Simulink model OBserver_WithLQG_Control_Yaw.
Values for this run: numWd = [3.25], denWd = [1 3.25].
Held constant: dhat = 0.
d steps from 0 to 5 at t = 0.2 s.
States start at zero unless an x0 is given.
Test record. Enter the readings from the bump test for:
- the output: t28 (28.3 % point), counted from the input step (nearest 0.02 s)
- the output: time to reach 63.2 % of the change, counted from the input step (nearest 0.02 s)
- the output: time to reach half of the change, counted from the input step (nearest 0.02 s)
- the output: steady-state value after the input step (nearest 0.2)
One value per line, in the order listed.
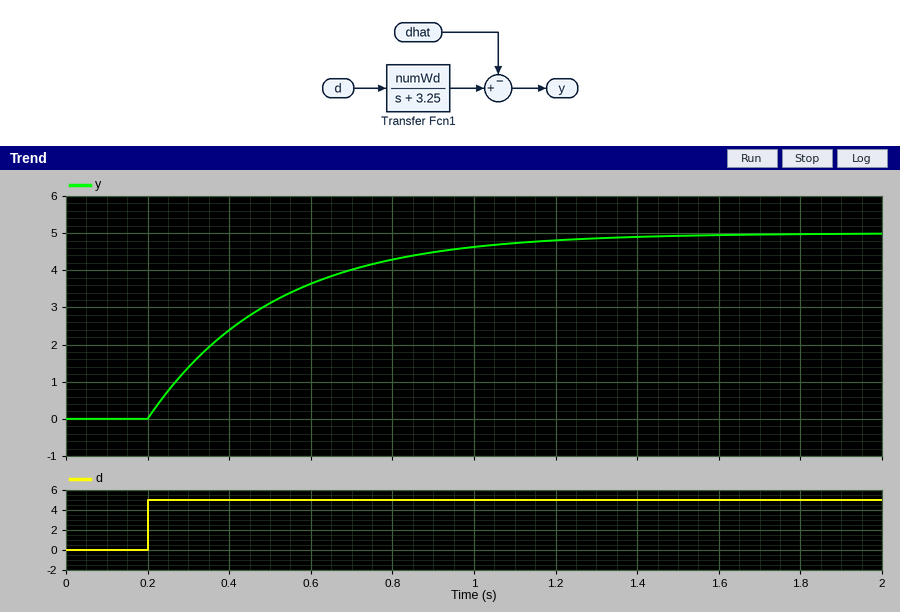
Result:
0.10 s
0.30 s
0.22 s
5.0
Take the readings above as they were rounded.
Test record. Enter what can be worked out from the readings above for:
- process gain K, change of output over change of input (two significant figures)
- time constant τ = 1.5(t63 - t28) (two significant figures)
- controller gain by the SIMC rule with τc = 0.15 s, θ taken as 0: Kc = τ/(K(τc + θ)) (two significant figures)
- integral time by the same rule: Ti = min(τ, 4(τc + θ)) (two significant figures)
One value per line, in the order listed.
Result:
1.0
0.30 s
2.0
0.30 s
